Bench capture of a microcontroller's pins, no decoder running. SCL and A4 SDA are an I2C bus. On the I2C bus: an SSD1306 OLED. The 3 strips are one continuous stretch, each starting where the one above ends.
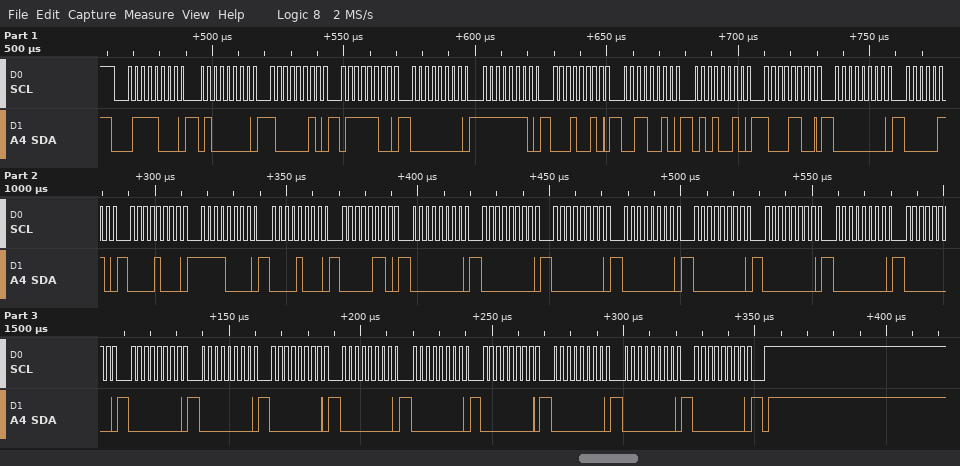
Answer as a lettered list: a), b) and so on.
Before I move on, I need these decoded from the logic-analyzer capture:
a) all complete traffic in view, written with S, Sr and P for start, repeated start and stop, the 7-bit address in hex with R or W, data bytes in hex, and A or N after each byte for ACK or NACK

a) S 3CW A 40 A 82 A 7C A 00 A FE A 12 A 32 A 52 A 8C A 00 A 06 A 08 A F0 A 08 A 06 A 00 A 00 A 00 A 00 A 00 A 00 A 00 A 00 A 00 A 00 A 00 A 00 A 00 A 00 A 00 A 00 A 00 A P
